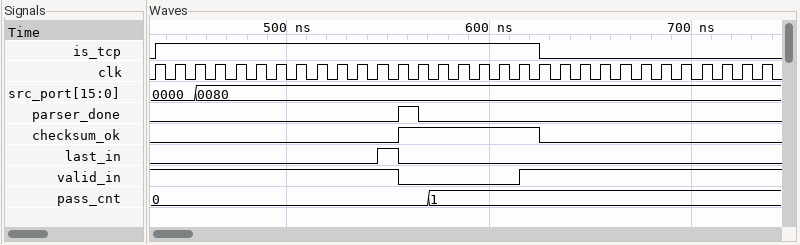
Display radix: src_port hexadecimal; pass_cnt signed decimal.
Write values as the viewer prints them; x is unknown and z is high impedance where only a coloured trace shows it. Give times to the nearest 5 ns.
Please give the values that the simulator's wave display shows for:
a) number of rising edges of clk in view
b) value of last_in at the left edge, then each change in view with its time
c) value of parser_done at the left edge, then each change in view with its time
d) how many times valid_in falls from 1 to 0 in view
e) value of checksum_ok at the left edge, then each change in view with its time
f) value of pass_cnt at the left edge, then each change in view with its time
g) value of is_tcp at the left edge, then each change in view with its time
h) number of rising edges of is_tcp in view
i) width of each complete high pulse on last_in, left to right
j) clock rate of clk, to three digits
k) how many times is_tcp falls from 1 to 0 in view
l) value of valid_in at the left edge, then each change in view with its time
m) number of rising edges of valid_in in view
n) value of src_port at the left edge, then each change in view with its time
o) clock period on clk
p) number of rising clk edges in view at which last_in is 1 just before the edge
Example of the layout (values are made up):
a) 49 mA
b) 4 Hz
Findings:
a) 31
b) 0, 1 at 545 ns, 0 at 555 ns
c) 0, 1 at 555 ns, 0 at 565 ns
d) 1
e) 0, 1 at 555 ns, 0 at 625 ns
f) 0, 1 at 570 ns
g) 0, 1 at 435 ns, 0 at 625 ns
h) 1
i) 10 ns
j) 100 MHz
k) 1
l) 1, 0 at 555 ns, 1 at 615 ns
m) 1
n) 0000, 0080 at 455 ns
o) 10 ns
p) 1
